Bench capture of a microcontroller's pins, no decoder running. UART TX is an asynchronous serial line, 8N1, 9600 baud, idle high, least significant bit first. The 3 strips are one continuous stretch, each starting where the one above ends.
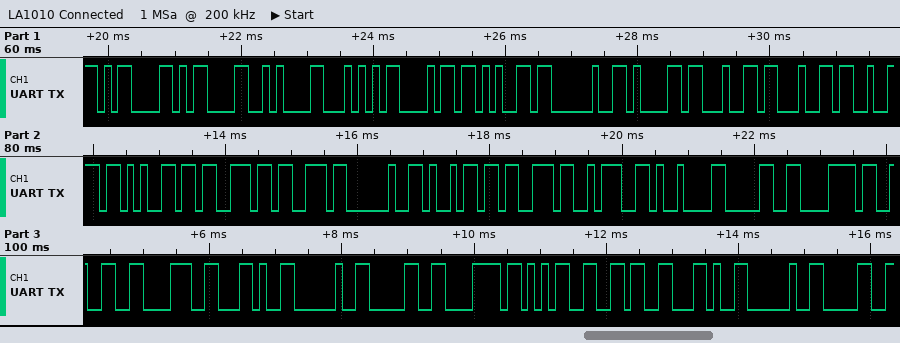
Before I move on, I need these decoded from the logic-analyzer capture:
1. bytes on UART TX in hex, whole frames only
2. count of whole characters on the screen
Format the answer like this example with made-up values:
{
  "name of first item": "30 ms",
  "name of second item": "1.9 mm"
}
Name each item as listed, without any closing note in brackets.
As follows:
{
  "bytes on UART TX in hex, whole frames only": "0x0D 0x0D 0x0A 0x54 0x68 0x65 0x20 0x61 0x64 0x64 0x72 0x65 0x73 0x73 0x20 0x69 0x73 0x3A 0x09 0x30 0x78 0x32 0x38 0x2C 0x20 0x30 0x78 0x35 0x36 0x2C 0x20 0x30",
  "count of whole characters on the screen": "32"
}
